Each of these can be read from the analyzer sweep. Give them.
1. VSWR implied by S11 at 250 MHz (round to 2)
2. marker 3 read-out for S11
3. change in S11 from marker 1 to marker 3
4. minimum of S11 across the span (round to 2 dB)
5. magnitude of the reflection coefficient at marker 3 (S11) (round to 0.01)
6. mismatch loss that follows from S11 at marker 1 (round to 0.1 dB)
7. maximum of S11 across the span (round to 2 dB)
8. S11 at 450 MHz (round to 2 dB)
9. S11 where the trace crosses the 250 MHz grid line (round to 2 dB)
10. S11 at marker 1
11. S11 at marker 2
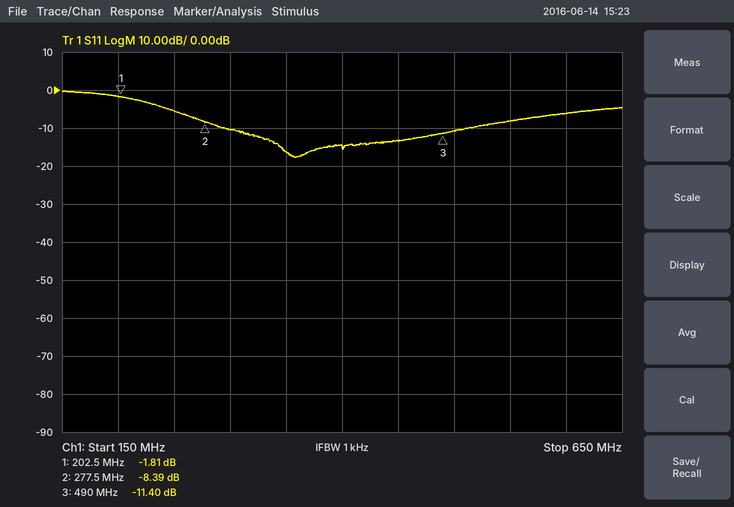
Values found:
4
-11.40 dB
-9.59 dB
-18 dB
0.27
4.7 dB
0 dB
-14 dB
-6 dB
-1.81 dB
-8.39 dB
